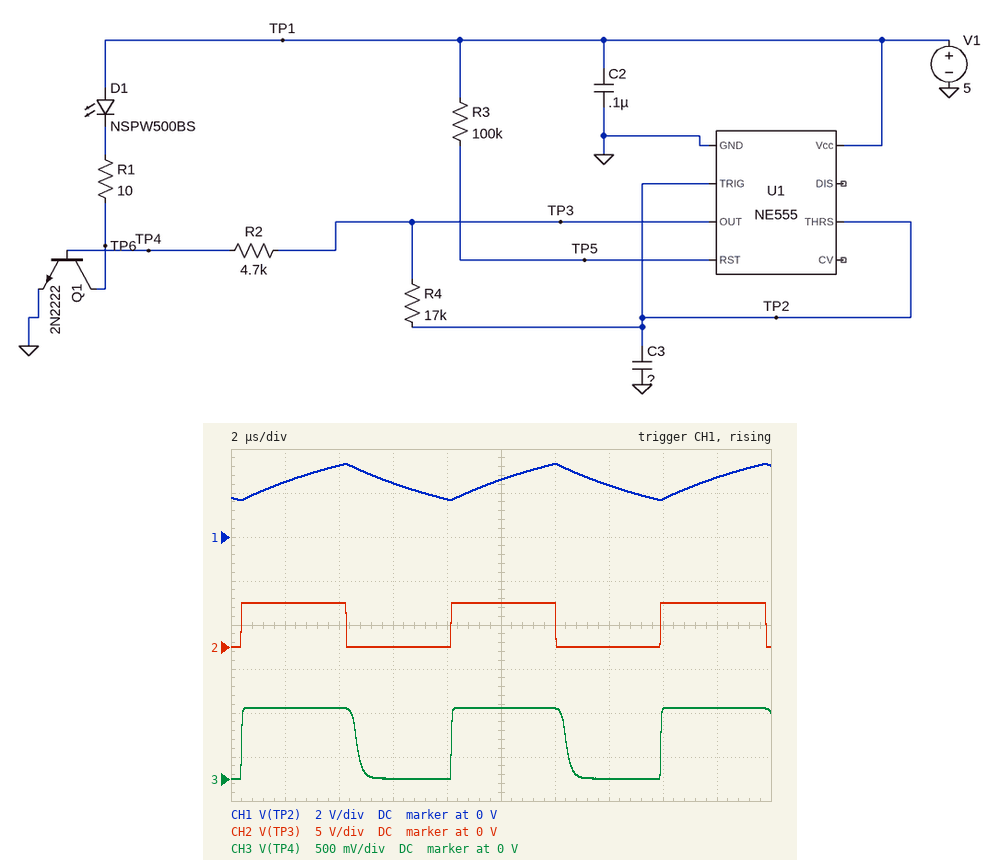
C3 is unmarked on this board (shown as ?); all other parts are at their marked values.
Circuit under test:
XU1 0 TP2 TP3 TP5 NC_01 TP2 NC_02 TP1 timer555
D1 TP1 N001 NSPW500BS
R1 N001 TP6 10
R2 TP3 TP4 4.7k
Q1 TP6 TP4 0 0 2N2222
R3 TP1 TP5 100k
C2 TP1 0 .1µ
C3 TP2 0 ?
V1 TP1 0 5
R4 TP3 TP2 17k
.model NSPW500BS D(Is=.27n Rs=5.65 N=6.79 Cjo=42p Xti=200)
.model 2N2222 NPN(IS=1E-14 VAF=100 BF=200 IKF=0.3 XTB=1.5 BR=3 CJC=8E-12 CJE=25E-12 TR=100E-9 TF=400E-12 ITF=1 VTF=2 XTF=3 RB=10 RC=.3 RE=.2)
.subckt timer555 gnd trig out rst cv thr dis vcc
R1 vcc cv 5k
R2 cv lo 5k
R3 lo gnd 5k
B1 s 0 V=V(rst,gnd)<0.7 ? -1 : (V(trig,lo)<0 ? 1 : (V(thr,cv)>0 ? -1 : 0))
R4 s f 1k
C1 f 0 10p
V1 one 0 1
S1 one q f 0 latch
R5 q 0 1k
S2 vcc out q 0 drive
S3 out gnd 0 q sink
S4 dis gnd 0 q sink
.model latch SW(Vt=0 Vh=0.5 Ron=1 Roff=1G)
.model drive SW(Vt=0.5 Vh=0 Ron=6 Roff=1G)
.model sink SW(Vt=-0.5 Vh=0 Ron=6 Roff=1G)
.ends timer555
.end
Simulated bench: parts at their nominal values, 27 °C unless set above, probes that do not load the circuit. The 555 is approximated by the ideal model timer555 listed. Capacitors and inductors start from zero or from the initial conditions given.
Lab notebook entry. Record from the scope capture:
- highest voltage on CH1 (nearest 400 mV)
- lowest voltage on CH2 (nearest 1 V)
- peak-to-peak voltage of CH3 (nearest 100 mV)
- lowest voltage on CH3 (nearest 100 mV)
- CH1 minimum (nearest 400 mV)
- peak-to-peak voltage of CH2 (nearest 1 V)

3.2 V
0 V
800 mV
0 V
1.6 V
5 V
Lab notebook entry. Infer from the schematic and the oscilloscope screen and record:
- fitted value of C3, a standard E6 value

330 pF
